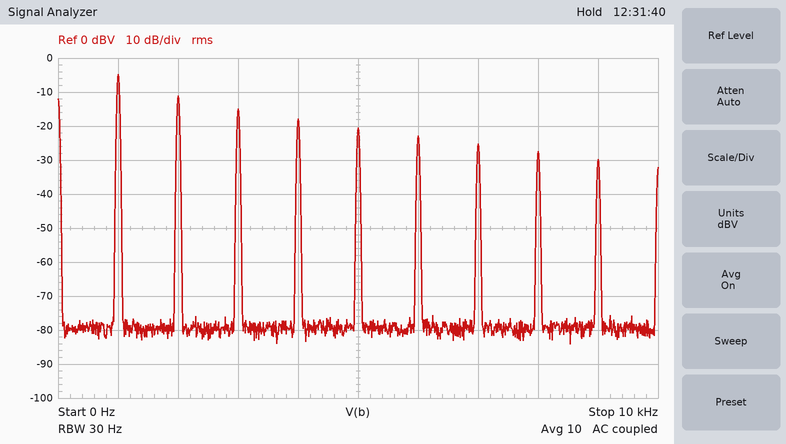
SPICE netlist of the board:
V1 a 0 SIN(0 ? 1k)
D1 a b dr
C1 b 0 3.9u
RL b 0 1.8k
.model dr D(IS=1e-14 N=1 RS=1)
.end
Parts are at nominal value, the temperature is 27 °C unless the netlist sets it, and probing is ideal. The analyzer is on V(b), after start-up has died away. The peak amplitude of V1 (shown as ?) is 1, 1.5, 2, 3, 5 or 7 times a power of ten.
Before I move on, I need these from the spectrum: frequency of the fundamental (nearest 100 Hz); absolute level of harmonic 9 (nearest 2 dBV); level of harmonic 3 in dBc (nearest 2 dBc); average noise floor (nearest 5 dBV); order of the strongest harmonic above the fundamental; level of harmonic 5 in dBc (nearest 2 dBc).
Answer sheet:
1.0 kHz
-30 dBV
-10 dBc
-80 dBV
2
-16 dBc
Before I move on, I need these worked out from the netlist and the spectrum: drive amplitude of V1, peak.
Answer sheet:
20 V
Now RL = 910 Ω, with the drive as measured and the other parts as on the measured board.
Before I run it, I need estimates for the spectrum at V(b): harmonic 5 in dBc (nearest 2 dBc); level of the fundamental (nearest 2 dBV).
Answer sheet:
-18 dBc
0 dBV
